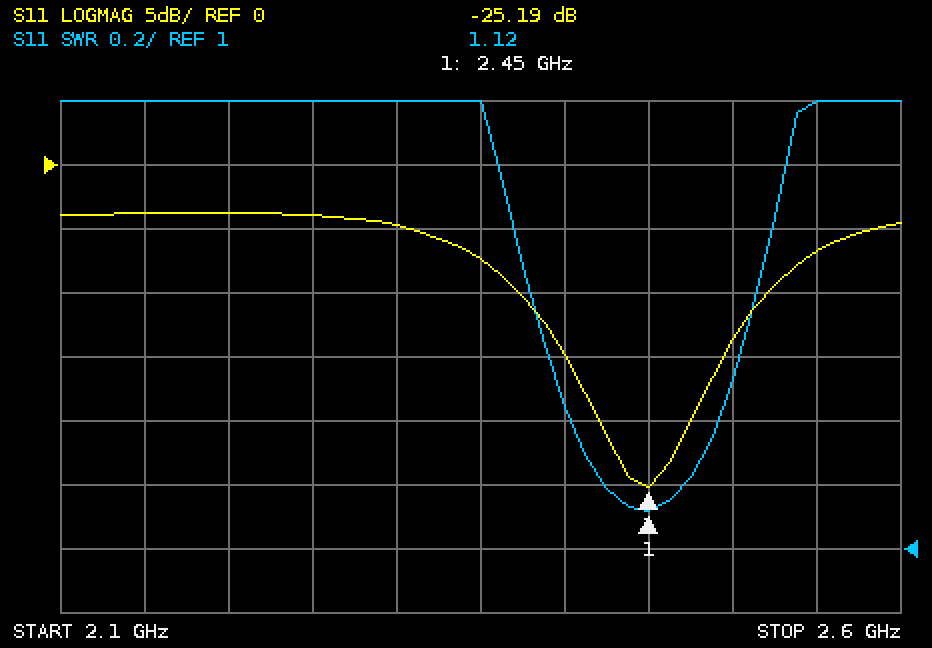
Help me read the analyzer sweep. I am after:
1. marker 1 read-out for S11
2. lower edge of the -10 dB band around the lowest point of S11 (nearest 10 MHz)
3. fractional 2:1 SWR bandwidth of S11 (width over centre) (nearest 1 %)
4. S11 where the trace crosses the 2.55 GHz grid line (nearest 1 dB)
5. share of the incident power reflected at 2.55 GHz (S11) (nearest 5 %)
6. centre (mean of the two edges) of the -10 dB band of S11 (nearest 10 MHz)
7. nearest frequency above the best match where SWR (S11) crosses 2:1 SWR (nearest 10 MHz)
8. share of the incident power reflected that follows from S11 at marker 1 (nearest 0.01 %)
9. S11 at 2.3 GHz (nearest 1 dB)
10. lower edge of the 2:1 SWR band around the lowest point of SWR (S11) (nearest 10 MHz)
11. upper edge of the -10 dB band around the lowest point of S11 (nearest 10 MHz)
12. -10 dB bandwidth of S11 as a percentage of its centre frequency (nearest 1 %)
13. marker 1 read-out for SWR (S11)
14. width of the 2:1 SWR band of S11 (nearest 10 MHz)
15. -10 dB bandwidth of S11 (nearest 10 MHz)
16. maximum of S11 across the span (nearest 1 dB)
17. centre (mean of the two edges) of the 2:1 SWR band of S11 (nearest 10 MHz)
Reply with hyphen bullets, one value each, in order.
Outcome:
- -25.19 dB
- 2.37 GHz
- 6 %
- -7 dB
- 20 %
- 2.45 GHz
- 2.52 GHz
- 0.30 %
- -5 dB
- 2.37 GHz
- 2.52 GHz
- 6 %
- 1.12
- 150 MHz
- 150 MHz
- -4 dB
- 2.45 GHz
